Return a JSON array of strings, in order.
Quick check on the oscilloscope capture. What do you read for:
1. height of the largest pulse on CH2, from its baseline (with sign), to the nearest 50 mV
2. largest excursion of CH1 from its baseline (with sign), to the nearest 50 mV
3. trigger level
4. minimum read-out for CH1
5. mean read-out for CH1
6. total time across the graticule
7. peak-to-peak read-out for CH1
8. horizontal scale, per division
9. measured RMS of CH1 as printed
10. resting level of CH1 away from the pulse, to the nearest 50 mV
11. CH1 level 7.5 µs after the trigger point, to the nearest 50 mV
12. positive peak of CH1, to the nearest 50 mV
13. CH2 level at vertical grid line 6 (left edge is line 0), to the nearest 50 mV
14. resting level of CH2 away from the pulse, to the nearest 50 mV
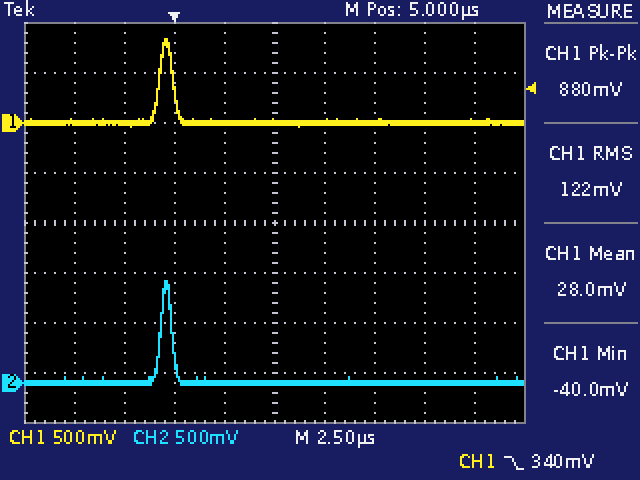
["+1.00 V", "+850 mV", "340 mV", "-40.0 mV", "28.0 mV", "25 µs", "880 mV", "2.5 µs", "122 mV", "0 mV", "0 mV", "850 mV", "0 mV", "0 mV"]
